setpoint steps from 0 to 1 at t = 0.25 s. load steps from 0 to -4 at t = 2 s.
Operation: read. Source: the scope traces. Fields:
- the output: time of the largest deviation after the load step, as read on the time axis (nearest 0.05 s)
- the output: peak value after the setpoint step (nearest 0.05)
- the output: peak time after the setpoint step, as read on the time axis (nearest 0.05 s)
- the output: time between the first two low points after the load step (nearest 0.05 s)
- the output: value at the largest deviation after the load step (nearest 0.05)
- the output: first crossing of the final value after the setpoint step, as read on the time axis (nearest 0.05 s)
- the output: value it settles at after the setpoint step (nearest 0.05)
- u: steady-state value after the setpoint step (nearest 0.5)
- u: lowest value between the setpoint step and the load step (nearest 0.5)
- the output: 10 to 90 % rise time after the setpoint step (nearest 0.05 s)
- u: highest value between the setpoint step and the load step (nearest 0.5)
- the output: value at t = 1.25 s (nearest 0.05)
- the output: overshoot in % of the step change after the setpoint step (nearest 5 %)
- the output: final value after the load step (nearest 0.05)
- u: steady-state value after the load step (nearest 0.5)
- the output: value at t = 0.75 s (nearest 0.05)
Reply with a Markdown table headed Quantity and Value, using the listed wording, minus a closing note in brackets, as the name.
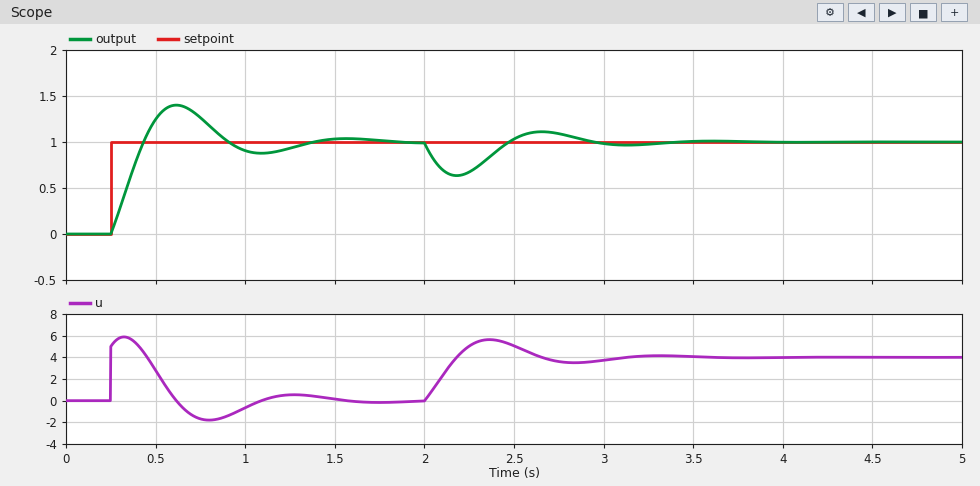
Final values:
| Quantity | Value |
|---|---|
| the output: time of the largest deviation after the load step, as read on the time axis | 2.20 s |
| the output: peak value after the setpoint step | 1.40 |
| the output: peak time after the setpoint step, as read on the time axis | 0.60 s |
| the output: time between the first two low points after the load step | 0.95 s |
| the output: value at the largest deviation after the load step | 0.65 |
| the output: first crossing of the final value after the setpoint step, as read on the time axis | 0.45 s |
| the output: value it settles at after the setpoint step | 1.00 |
| u: steady-state value after the setpoint step | 0.0 |
| u: lowest value between the setpoint step and the load step | -2.0 |
| the output: 10 to 90 % rise time after the setpoint step | 0.15 s |
| u: highest value between the setpoint step and the load step | 6.0 |
| the output: value at t = 1.25 s | 0.95 |
| the output: overshoot in % of the step change after the setpoint step | 40 % |
| the output: final value after the load step | 1.00 |
| u: steady-state value after the load step | 4.0 |
| the output: value at t = 0.75 s | 1.25 |
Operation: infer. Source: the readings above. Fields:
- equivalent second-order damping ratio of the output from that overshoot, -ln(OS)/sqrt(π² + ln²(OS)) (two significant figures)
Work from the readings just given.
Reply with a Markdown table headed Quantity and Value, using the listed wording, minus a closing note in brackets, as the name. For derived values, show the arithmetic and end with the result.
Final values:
| Quantity | Value |
|---|---|
| equivalent second-order damping ratio of the output from that overshoot, -ln(OS)/sqrt(π² + ln²(OS)) | ln(0.4) = -0.916; 0.916 / sqrt(9.870 + 0.840) = 0.28 |
